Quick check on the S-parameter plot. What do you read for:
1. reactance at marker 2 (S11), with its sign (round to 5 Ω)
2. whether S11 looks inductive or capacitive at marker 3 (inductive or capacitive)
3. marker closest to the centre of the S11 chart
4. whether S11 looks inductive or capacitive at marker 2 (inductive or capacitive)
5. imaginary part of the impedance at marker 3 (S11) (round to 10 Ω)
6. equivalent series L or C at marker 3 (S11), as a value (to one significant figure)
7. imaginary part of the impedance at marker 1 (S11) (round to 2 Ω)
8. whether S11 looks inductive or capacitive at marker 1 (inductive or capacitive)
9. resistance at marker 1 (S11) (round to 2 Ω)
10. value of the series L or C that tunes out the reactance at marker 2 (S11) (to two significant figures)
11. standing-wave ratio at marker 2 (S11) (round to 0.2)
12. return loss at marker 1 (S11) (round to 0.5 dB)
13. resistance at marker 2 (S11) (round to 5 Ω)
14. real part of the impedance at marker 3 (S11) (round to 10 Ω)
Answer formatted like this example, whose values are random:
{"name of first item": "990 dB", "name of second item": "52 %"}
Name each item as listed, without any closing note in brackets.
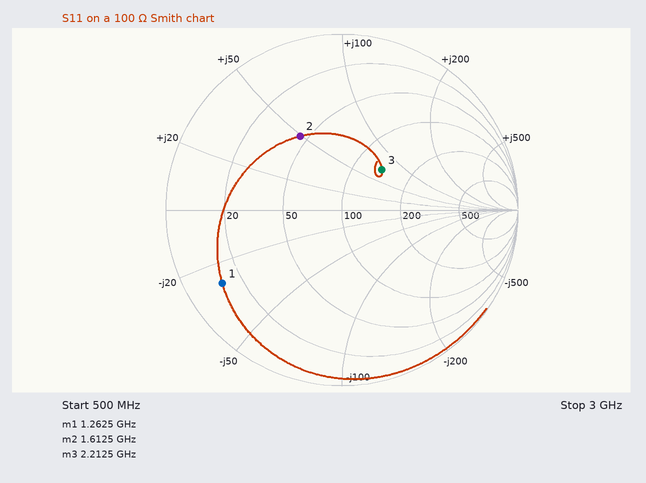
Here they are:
{"reactance at marker 2 (S11), with its sign": "+50 Ω", "whether S11 looks inductive or capacitive at marker 3": "inductive", "marker closest to the centre of the S11 chart": "marker 3", "whether S11 looks inductive or capacitive at marker 2": "inductive", "imaginary part of the impedance at marker 3 (S11)": "+70 Ω", "equivalent series L or C at marker 3 (S11), as a value": "5 nH", "imaginary part of the impedance at marker 1 (S11)": "-28 Ω", "whether S11 looks inductive or capacitive at marker 1": "capacitive", "resistance at marker 1 (S11)": "12 Ω", "value of the series L or C that tunes out the reactance at marker 2 (S11)": "2.0 pF", "standing-wave ratio at marker 2 (S11)": "2.8", "return loss at marker 1 (S11)": "2.0 dB", "resistance at marker 2 (S11)": "45 Ω", "real part of the impedance at marker 3 (S11)": "140 Ω"}
